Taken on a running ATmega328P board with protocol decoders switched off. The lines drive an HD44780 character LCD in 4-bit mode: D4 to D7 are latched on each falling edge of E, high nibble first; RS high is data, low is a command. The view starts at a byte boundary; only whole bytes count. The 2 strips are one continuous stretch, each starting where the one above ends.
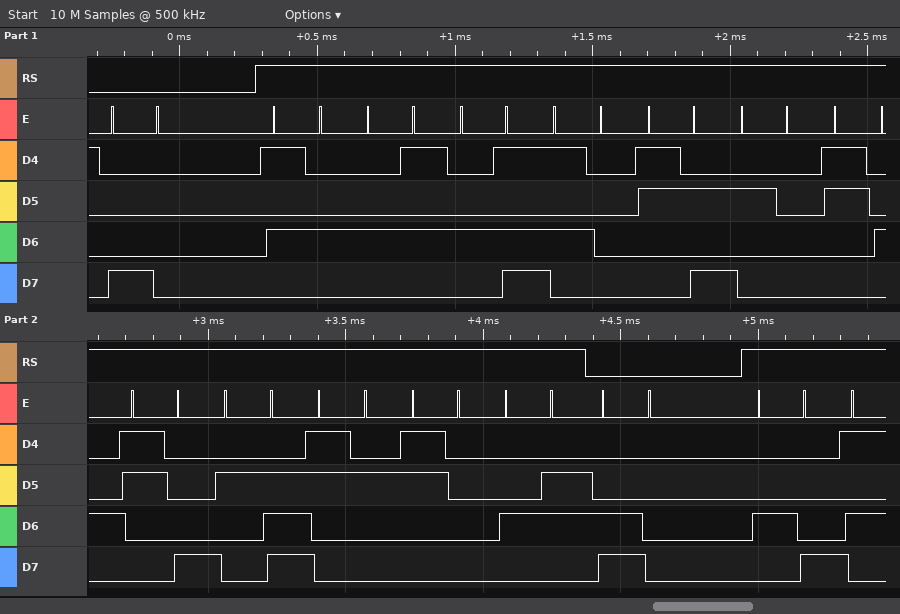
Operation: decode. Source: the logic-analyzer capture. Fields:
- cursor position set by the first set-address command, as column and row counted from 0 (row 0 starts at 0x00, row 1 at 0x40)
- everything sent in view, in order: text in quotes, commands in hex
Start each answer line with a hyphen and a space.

- column 0, row 0
- 0x80 "TEMP: 48.20F" 0xC0 "H"
